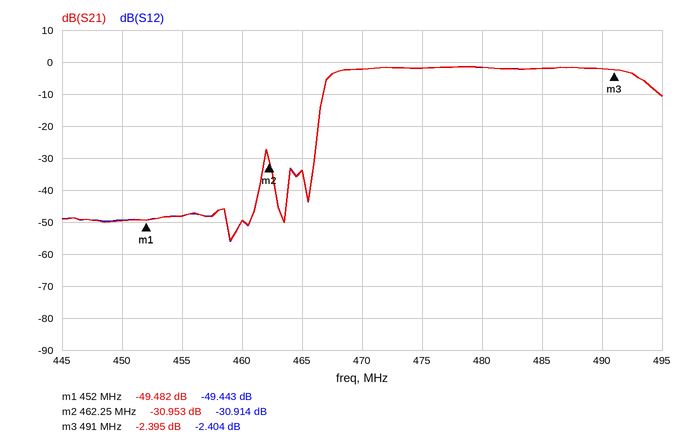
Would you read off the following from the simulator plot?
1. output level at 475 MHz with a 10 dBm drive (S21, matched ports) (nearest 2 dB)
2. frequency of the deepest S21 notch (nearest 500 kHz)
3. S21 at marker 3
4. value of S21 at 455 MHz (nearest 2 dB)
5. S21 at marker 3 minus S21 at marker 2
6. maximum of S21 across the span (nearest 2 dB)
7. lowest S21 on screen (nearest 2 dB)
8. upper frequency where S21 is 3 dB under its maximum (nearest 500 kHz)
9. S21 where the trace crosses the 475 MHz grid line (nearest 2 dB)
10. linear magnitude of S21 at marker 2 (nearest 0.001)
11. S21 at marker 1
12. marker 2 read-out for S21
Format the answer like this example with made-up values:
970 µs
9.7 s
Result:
8 dBm
459.0 MHz
-2.395 dB
-48 dB
28.558 dB
-2 dB
-56 dB
493.0 MHz
-2 dB
0.028
-49.482 dB
-30.953 dB
